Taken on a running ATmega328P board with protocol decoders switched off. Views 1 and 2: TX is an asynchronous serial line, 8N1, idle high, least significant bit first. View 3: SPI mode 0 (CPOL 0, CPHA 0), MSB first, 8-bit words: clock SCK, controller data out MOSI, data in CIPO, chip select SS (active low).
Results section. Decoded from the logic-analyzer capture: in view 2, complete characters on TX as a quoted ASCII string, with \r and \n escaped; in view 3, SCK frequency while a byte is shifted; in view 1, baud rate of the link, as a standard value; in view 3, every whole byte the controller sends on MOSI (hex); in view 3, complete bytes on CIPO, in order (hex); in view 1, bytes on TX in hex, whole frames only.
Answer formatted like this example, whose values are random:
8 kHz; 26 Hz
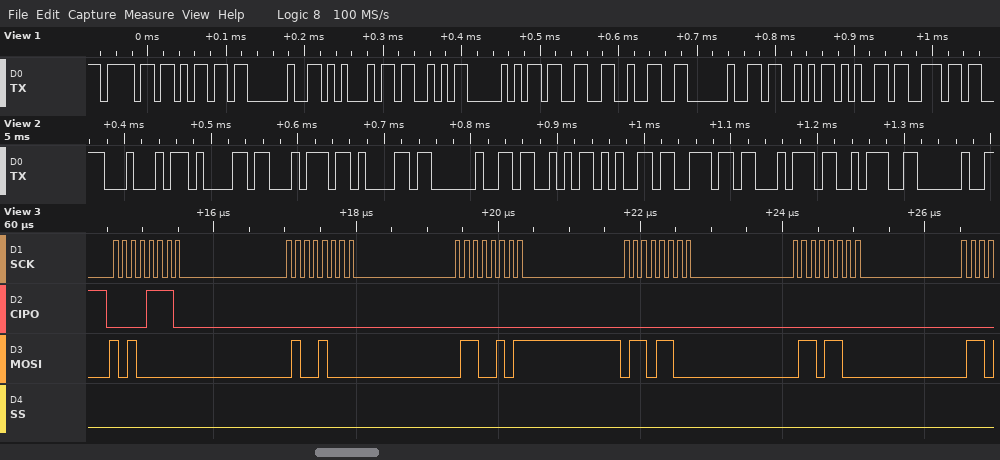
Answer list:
"Data Sent: "; 8 MHz; 115200 baud; A0 48 65 6C 6C; 0E 00 00 00 00; 6F 6D 20 45 53 50 33 32 20 53 65 6E
